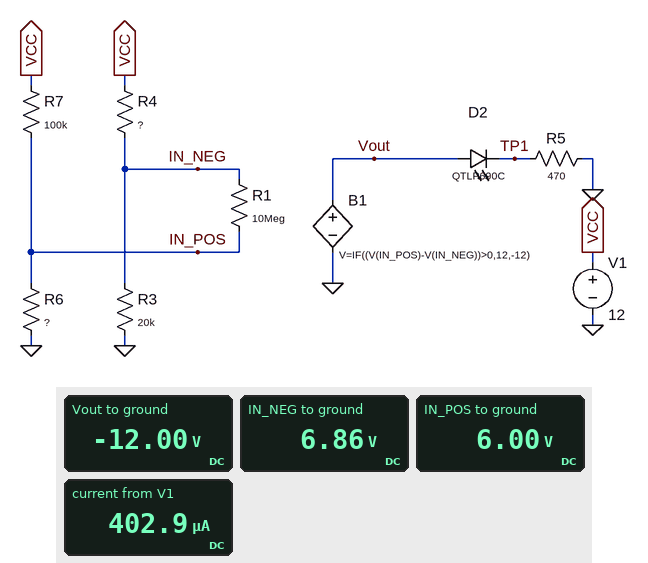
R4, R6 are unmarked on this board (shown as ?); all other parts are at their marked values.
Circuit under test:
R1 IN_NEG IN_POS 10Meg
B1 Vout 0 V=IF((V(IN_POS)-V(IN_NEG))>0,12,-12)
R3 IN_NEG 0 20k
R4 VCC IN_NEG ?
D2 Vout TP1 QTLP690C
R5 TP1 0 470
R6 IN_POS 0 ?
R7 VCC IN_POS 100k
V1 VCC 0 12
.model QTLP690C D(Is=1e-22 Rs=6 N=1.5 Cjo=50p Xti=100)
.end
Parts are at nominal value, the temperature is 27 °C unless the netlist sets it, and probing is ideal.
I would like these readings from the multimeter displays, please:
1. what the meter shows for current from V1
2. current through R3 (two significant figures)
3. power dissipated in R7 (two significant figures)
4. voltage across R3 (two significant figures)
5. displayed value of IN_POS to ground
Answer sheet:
402.9 µA
340 µA
360 µW
6.9 V
6.00 V
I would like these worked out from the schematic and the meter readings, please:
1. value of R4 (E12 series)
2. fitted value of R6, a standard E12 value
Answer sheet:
15 kΩ
100 kΩ
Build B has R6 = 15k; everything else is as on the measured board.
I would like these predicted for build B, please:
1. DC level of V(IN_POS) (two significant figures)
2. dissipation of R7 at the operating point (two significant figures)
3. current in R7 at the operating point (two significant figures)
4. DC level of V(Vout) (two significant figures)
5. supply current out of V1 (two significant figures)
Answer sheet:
1.6 V
1.1 mW
100 µA
-12 V
450 µA
